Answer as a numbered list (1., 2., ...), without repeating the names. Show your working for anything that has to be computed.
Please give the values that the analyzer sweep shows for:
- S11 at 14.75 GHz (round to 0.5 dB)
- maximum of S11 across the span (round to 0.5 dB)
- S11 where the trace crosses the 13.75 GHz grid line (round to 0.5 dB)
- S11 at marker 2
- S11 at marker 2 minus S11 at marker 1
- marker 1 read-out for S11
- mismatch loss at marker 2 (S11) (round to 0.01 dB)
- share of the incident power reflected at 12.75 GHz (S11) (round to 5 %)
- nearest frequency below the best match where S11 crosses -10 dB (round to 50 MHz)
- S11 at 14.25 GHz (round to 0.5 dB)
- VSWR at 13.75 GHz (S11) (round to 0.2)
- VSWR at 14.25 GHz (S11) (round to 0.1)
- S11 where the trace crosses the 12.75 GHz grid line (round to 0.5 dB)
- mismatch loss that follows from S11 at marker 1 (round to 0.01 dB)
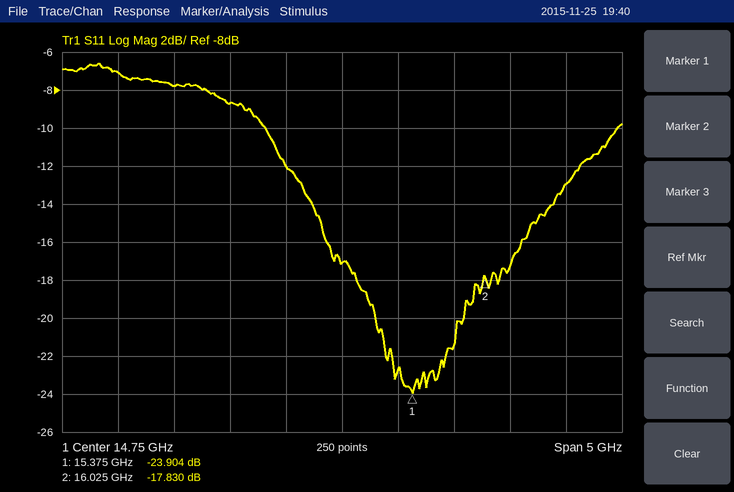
1. -17.0 dB
2. -6.5 dB
3. -8.5 dB
4. -17.830 dB
5. -17.83 − (-23.904) = 6.074 dB
6. -23.904 dB
7. −10 log10(1 − 10^(-17.83/10)) ≈ 0.07 dB
8. 10^(-7/10) ≈ 20 %
9. 14.05 GHz
10. -12.0 dB
11. |Γ| = 10^(-8.5/20) = 0.3758; VSWR = (1 + 0.3758)/(1 − 0.3758) ≈ 2.2
12. |Γ| = 10^(-12/20) = 0.2512; VSWR = (1 + 0.2512)/(1 − 0.2512) ≈ 1.7
13. -7.0 dB
14. −10 log10(1 − 10^(-23.904/10)) ≈ 0.02 dB
